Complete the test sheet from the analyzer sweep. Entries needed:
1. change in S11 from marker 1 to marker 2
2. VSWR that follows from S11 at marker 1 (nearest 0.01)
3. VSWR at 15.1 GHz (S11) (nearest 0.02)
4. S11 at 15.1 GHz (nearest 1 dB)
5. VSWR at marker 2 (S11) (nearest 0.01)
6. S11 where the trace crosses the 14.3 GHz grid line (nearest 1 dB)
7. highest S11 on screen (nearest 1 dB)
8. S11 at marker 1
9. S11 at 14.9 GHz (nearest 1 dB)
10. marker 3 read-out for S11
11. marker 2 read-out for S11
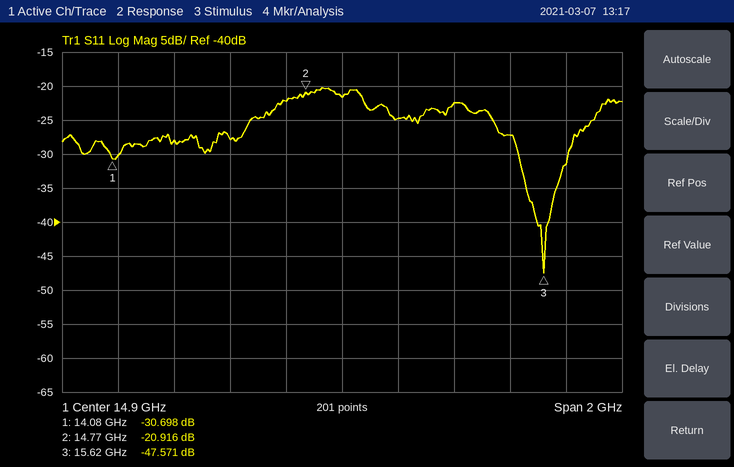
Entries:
9.782 dB
1.06
1.12
-25 dB
1.20
-28 dB
-20 dB
-30.698 dB
-22 dB
-47.571 dB
-20.916 dB
